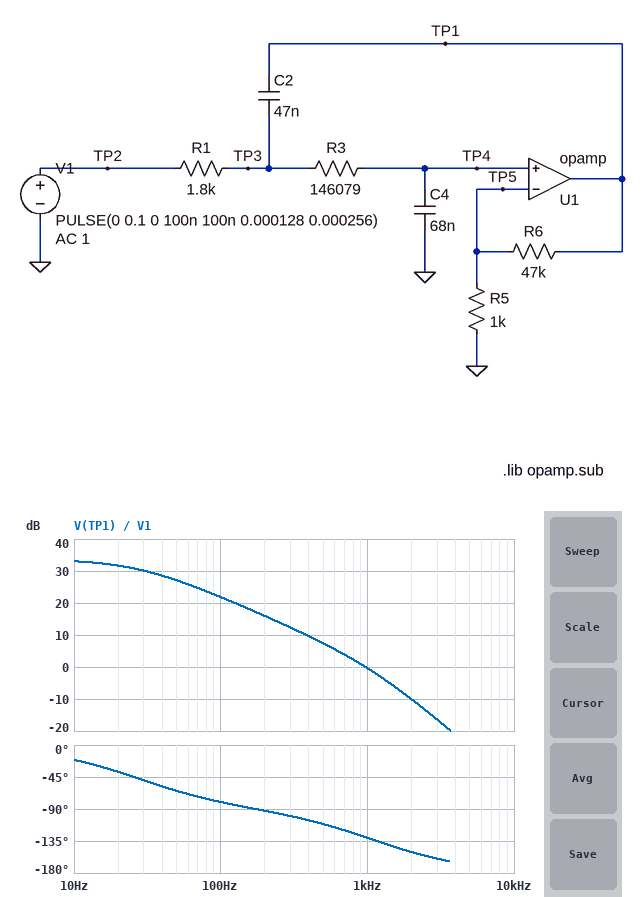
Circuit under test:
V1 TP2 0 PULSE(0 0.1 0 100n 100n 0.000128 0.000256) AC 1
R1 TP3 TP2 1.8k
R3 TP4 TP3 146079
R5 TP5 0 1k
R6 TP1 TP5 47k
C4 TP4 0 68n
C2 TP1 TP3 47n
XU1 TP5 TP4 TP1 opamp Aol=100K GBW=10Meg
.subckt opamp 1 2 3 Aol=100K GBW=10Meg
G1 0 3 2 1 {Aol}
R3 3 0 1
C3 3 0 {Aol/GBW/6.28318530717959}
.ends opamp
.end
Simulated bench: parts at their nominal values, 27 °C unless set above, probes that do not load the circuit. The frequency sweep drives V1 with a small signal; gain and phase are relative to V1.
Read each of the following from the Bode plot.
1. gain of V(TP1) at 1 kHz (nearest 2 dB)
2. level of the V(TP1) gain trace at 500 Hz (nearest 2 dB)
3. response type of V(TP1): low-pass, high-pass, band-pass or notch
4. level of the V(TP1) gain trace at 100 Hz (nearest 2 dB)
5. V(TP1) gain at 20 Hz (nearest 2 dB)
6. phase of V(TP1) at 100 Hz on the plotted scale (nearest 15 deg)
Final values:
0 dB
8 dB
low-pass
22 dB
32 dB
-75 deg
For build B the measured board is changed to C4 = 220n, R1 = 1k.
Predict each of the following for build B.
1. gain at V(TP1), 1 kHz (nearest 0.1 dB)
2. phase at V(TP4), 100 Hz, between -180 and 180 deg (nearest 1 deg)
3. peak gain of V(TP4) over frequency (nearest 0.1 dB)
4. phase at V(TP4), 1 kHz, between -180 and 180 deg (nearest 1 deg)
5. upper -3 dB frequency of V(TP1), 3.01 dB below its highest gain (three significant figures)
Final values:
-12.3 dB
-89 deg
0 dB
-107 deg
5.29 Hz
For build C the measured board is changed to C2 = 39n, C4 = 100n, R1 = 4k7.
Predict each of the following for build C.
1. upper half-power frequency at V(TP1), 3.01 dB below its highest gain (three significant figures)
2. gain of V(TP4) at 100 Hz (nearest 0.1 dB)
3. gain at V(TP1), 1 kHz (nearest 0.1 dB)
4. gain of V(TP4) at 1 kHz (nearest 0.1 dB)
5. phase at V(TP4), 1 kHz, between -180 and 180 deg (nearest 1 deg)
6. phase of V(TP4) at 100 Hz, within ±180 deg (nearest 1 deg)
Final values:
26.3 Hz
-12.2 dB
-7.4 dB
-41.0 dB
-159 deg
-91 deg
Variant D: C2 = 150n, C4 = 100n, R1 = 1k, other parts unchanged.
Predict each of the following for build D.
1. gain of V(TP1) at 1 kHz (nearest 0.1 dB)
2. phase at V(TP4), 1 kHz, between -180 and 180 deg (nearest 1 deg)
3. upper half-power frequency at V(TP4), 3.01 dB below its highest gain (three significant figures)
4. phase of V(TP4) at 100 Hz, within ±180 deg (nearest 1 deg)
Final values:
-6.2 dB
-151 deg
21.6 Hz
-88 deg
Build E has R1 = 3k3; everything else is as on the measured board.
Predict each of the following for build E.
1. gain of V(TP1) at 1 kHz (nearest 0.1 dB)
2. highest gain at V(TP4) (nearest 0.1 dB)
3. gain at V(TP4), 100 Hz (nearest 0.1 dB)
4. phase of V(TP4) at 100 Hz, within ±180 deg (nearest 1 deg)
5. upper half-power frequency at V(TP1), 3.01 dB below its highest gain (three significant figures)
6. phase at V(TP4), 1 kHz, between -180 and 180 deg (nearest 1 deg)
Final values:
-2.3 dB
0 dB
-5.3 dB
-78 deg
67.4 Hz
-163 deg
